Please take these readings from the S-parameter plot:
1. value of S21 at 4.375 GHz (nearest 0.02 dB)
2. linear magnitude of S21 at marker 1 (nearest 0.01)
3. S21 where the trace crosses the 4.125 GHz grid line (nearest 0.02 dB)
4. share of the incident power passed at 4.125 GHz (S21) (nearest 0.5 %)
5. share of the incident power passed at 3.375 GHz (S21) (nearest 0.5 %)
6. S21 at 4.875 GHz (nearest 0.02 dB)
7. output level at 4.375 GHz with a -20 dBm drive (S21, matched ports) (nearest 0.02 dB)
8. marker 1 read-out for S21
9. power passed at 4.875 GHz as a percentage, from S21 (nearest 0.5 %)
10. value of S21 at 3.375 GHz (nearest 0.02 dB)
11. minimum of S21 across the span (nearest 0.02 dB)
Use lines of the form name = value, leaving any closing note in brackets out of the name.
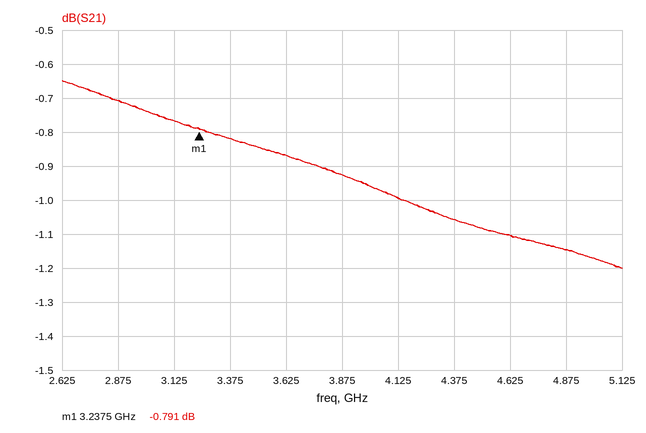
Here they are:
value of S21 at 4.375 GHz = -1.06 dB
linear magnitude of S21 at marker 1 = 0.91
S21 where the trace crosses the 4.125 GHz grid line = -1.00 dB
share of the incident power passed at 4.125 GHz (S21) = 79.5 %
share of the incident power passed at 3.375 GHz (S21) = 83.0 %
S21 at 4.875 GHz = -1.14 dB
output level at 4.375 GHz with a -20 dBm drive (S21, matched ports) = -21.06 dBm
marker 1 read-out for S21 = -0.791 dB
power passed at 4.875 GHz as a percentage, from S21 = 77.0 %
value of S21 at 3.375 GHz = -0.82 dB
minimum of S21 across the span = -1.20 dB
